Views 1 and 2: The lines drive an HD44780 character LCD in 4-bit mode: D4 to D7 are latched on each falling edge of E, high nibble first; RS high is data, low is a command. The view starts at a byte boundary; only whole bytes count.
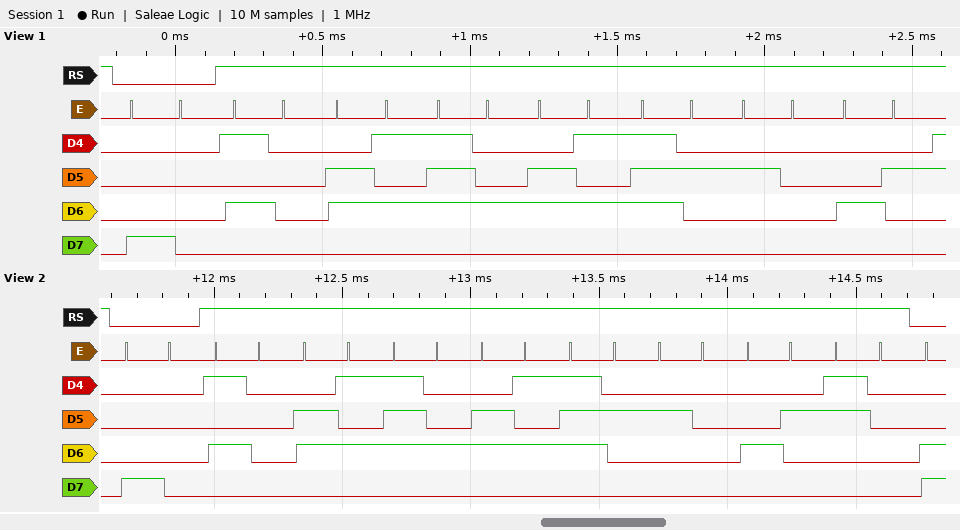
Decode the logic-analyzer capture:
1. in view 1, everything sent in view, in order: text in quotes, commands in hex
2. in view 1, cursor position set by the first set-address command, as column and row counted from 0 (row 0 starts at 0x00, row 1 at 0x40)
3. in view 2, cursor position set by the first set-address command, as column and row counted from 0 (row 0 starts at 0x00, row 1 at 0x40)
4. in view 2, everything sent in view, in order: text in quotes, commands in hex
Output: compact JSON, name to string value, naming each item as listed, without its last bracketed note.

{"in view 1, everything sent in view, in order: text in quotes, commands in hex": "0x80 \"Peter B\"", "in view 1, cursor position set by the first set-address command, as column and row counted from 0": "column 0, row 0", "in view 2, cursor position set by the first set-address command, as column and row counted from 0": "column 0, row 0", "in view 2, everything sent in view, in order: text in quotes, commands in hex": "0x80 \"Peter B0\""}
